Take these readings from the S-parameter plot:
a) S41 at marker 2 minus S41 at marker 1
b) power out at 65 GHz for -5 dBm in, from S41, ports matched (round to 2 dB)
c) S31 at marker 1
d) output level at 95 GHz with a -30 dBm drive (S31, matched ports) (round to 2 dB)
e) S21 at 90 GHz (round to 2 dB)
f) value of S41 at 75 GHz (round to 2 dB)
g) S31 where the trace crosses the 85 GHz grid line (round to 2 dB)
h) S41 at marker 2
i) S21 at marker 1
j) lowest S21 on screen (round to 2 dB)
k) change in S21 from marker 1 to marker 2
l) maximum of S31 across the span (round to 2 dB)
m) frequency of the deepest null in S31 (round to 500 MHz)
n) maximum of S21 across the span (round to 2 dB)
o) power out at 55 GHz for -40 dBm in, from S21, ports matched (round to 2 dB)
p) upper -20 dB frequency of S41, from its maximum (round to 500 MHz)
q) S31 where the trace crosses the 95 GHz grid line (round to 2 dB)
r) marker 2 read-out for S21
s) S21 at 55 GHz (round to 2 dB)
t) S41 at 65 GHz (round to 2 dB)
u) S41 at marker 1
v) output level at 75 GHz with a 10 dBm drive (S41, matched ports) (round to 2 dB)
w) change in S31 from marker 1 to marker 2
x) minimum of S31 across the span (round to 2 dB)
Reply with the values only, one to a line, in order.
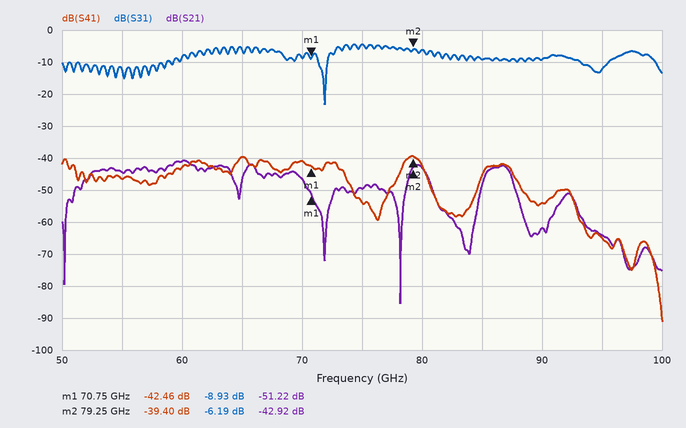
3.06 dB
-44 dBm
-8.93 dB
-42 dBm
-62 dB
-54 dB
-10 dB
-39.40 dB
-51.22 dB
-86 dB
8.30 dB
-4 dB
72.0 GHz
-40 dB
-84 dBm
93.0 GHz
-12 dB
-42.92 dB
-44 dB
-40 dB
-42.46 dB
-44 dBm
2.74 dB
-24 dB
